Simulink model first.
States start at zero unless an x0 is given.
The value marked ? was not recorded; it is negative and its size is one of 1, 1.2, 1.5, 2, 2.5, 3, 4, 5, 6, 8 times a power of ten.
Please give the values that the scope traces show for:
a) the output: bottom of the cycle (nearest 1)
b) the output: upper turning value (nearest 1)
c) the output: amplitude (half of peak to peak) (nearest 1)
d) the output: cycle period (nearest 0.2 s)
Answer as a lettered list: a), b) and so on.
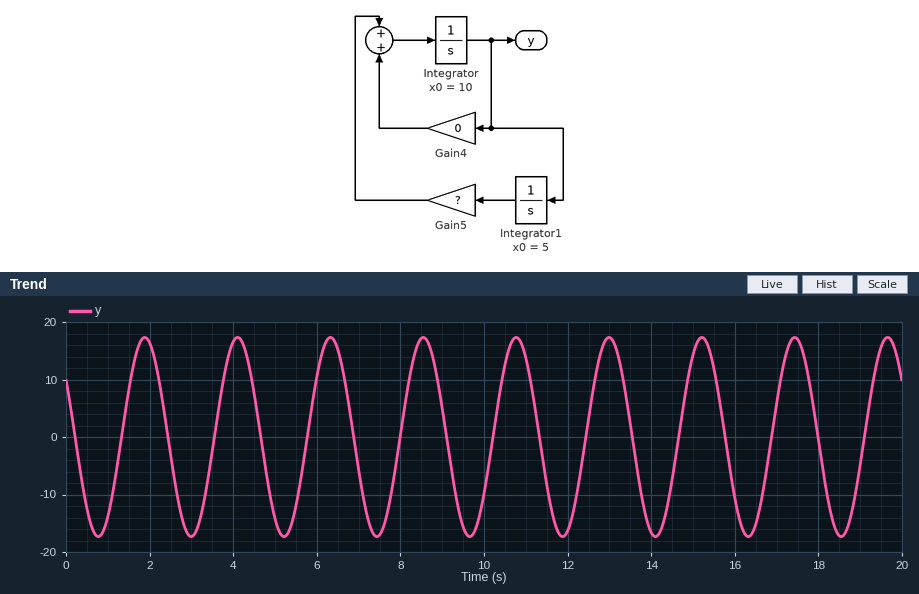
a) -17
b) 17
c) 17
d) 2.2 s
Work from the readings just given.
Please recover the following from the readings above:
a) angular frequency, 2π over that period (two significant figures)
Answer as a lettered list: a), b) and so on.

a) 2.9 rad/s
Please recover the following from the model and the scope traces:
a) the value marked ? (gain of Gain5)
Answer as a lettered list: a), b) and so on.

a) -8
